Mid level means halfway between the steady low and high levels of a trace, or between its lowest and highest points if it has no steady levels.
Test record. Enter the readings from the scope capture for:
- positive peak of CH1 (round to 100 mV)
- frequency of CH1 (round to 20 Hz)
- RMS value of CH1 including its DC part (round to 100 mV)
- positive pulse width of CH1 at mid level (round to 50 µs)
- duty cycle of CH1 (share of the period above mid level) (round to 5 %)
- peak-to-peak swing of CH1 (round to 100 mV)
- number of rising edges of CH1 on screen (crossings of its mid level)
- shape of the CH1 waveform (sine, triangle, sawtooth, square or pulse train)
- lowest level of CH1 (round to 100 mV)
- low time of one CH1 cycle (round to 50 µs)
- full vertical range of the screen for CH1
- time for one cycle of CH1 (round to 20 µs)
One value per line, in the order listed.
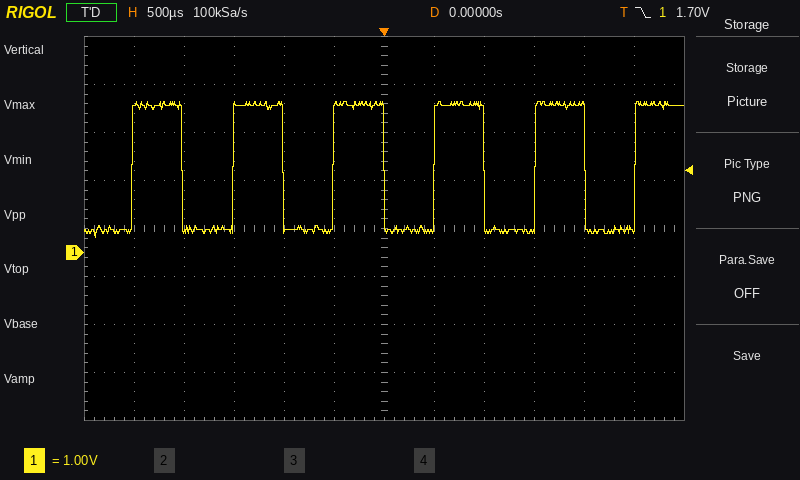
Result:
3.1 V
1.00 kHz
2.2 V
500 µs
50 %
2.8 V
6
square
300 mV
500 µs
8 V
1.00 ms
